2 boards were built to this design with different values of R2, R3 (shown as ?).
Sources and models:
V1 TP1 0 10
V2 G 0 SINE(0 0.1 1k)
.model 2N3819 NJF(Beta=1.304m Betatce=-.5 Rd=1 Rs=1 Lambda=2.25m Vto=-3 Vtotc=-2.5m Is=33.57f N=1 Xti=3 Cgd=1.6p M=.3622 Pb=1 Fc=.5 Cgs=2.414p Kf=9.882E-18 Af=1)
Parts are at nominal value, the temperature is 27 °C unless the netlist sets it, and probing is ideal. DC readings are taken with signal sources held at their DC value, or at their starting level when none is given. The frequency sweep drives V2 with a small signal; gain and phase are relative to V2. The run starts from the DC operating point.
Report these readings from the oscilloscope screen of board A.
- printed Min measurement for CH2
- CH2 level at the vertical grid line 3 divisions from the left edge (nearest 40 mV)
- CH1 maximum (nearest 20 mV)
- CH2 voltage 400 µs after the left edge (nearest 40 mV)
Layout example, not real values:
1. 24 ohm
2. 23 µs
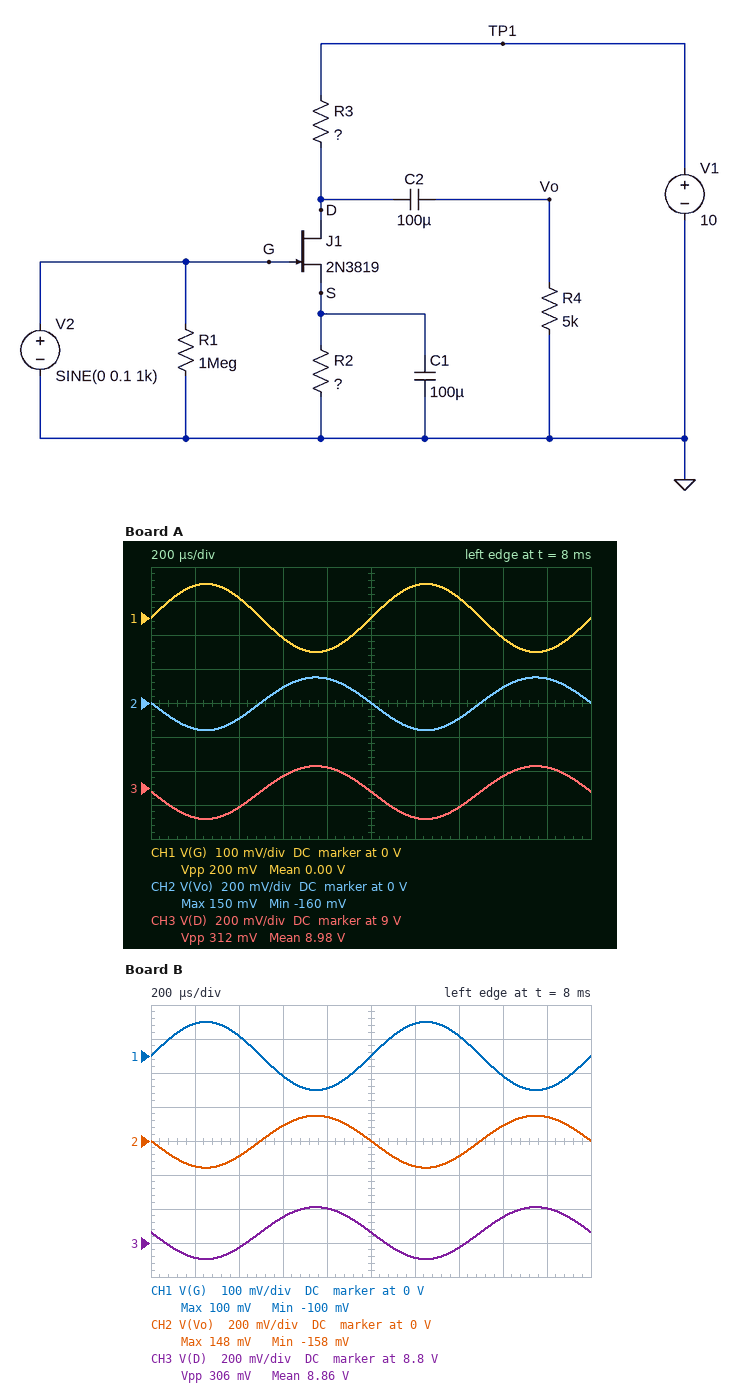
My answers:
1. -160 mV
2. 80 mV
3. 100 mV
4. -80 mV
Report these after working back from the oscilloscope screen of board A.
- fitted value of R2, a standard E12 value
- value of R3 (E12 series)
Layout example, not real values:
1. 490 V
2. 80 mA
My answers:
1. 1 kΩ
2. 560 Ω
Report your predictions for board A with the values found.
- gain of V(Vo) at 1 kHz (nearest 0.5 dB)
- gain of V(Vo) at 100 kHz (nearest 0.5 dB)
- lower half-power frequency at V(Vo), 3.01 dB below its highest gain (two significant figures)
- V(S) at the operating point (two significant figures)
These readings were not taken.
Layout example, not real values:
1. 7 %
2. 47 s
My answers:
1. 4.0 dB
2. 4.0 dB
3. 6.1 Hz
4. 1.8 V
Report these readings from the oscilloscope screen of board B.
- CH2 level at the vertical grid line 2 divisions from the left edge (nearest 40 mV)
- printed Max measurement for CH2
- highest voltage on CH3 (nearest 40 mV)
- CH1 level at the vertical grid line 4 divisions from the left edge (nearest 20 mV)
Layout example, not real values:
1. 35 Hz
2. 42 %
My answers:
1. -80 mV
2. 148 mV
3. 9.00 V
4. -100 mV
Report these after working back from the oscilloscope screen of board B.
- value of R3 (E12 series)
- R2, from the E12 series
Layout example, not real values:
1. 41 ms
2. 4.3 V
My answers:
1. 470 Ω
2. 680 Ω
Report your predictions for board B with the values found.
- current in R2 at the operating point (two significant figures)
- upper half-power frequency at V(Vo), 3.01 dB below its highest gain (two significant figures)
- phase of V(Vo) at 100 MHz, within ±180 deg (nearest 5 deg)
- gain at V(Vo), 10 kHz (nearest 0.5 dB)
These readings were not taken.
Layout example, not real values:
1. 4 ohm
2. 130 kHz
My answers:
1. 2.4 mA
2. 2.0 GHz
3. 165 deg
4. 3.5 dB
